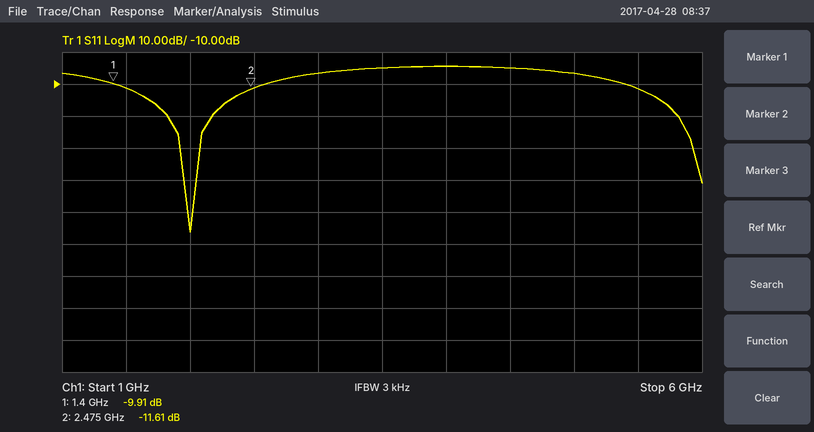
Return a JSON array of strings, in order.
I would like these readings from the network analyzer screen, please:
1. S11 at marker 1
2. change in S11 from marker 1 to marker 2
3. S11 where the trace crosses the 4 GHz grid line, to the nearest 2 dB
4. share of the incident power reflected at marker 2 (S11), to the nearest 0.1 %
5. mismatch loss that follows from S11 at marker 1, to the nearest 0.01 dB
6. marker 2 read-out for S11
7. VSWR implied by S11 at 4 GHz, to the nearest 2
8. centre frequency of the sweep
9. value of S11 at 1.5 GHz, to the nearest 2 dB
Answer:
["-9.91 dB", "-1.70 dB", "-4 dB", "6.9 %", "0.47 dB", "-11.61 dB", "4", "3.5 GHz", "-12 dB"]
